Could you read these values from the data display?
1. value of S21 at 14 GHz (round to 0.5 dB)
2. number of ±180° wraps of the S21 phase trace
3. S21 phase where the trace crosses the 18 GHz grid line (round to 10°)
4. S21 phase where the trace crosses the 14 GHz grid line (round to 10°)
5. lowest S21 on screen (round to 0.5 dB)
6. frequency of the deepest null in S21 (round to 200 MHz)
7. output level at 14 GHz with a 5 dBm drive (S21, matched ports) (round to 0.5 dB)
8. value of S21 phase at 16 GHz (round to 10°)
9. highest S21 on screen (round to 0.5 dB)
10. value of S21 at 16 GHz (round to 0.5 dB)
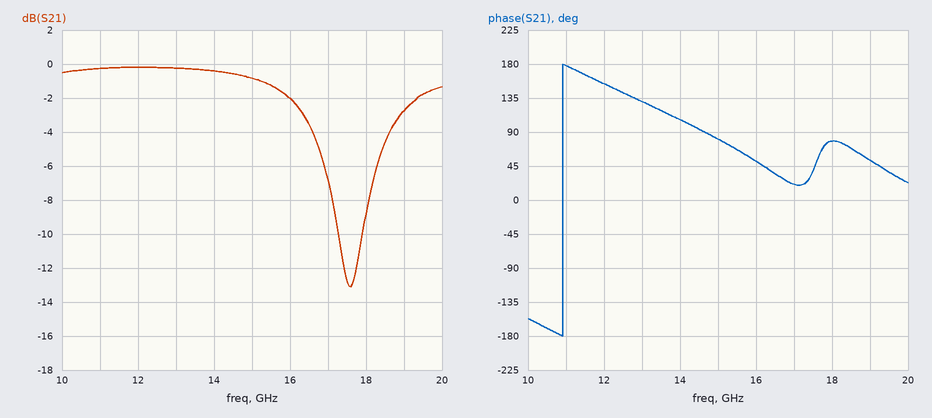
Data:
-0.5 dB
1
80°
110°
-13.0 dB
17.6 GHz
4.5 dBm
50°
0.0 dB
-2.0 dB
